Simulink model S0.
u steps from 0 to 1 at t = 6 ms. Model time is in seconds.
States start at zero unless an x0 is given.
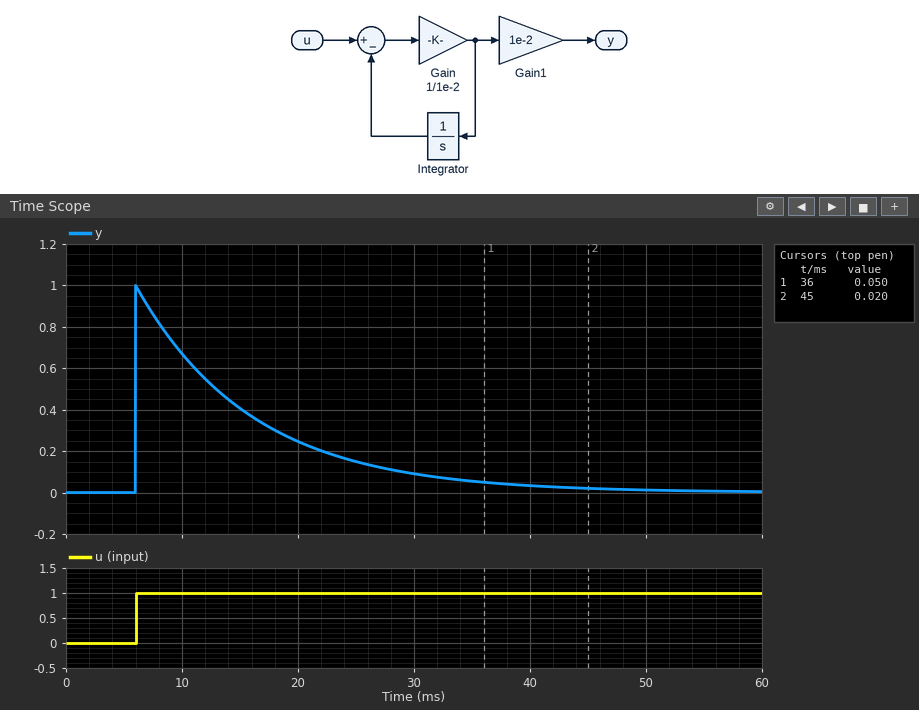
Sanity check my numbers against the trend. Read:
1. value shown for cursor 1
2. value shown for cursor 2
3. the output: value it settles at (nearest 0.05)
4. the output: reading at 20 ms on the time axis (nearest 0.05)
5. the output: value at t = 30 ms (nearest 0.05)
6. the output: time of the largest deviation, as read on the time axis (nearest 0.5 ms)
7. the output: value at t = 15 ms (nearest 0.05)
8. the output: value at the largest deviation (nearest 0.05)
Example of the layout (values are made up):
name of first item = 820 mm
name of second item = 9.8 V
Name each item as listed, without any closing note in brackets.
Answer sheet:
value shown for cursor 1 = 0.050
value shown for cursor 2 = 0.020
the output: value it settles at = 0.00
the output: reading at 20 ms on the time axis = 0.25
the output: value at t = 30 ms = 0.10
the output: time of the largest deviation, as read on the time axis = 6.0 ms
the output: value at t = 15 ms = 0.40
the output: value at the largest deviation = 1.00
